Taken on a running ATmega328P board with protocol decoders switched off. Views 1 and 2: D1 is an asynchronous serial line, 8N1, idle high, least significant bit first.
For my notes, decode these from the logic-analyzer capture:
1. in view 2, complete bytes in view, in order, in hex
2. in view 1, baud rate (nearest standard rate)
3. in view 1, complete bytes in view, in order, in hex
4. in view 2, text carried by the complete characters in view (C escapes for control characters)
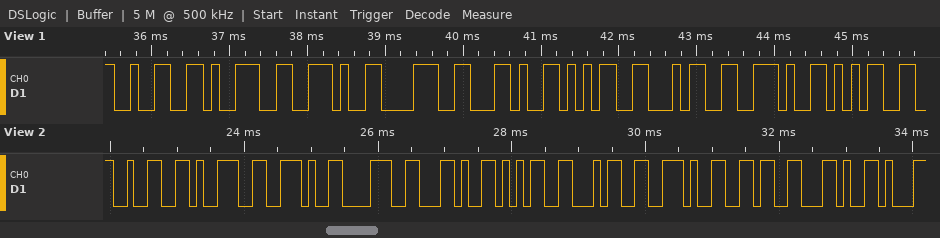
32 39 2E 38 2C 35 34 2E 36 2C
9600 baud
0x32 0x39 0x2E 0x38 0x2C 0x35 0x34 0x2E 0x35
"29.8,54.6,"
